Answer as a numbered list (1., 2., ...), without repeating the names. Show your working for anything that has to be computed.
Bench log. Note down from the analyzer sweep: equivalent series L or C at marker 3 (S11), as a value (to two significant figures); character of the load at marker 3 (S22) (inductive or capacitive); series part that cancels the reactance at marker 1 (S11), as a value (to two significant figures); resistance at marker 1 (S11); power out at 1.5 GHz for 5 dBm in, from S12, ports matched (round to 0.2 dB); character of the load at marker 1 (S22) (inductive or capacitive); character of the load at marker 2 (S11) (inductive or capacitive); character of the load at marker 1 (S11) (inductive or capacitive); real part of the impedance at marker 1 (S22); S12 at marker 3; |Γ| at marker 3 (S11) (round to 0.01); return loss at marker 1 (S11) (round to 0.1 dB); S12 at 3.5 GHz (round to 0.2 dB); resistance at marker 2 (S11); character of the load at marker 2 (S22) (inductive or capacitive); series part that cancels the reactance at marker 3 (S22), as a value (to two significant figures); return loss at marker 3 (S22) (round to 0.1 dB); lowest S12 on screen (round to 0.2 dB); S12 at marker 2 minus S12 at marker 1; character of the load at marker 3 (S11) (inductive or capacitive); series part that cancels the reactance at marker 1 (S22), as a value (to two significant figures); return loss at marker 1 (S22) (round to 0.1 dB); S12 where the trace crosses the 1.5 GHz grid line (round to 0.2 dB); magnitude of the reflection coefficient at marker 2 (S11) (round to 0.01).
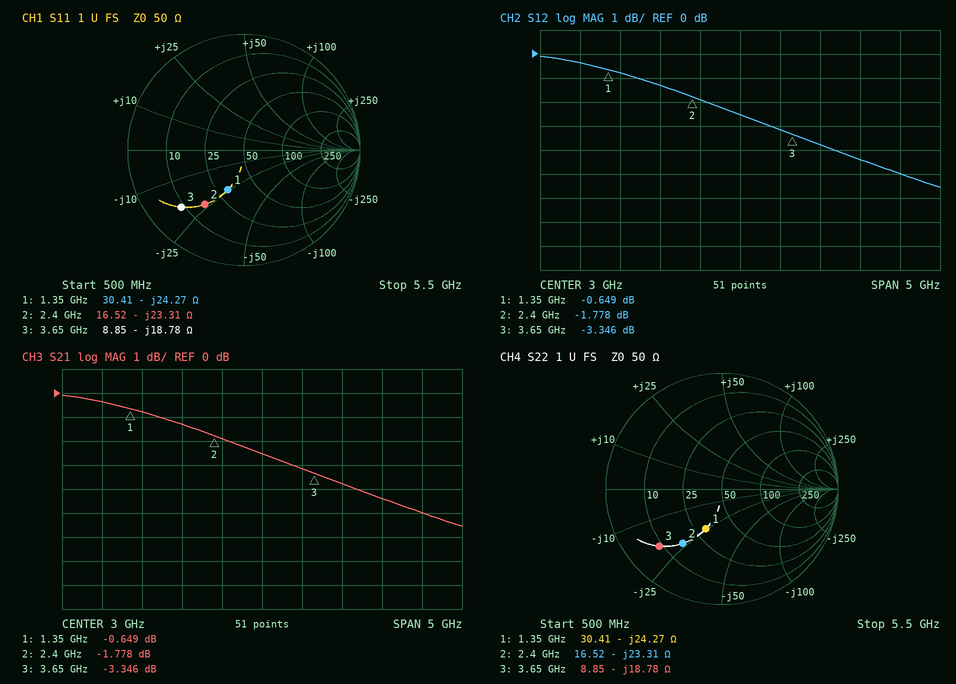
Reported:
1. C = 1/(2π × 3.65 GHz × 18.78 Ω) ≈ 2.3 pF
2. capacitive
3. L = 24.27 Ω/(2π × 1.35 GHz) ≈ 2.9 nH
4. 30.41 Ω
5. 5 dBm + (-0.8 dB) = 4.2 dBm
6. capacitive
7. capacitive
8. capacitive
9. 30.41 Ω
10. -3.346 dB
11. 0.73
12. 8.6 dB
13. -3.2 dB
14. 16.52 Ω
15. capacitive
16. L = 18.78 Ω/(2π × 3.65 GHz) ≈ 819 pH, so 820 pH to two significant figures
17. 2.7 dB
18. -5.6 dB
19. -1.778 − (-0.649) = -1.129 dB
20. capacitive
21. L = 24.27 Ω/(2π × 1.35 GHz) ≈ 2.9 nH
22. 8.6 dB
23. -0.8 dB
24. 0.58
